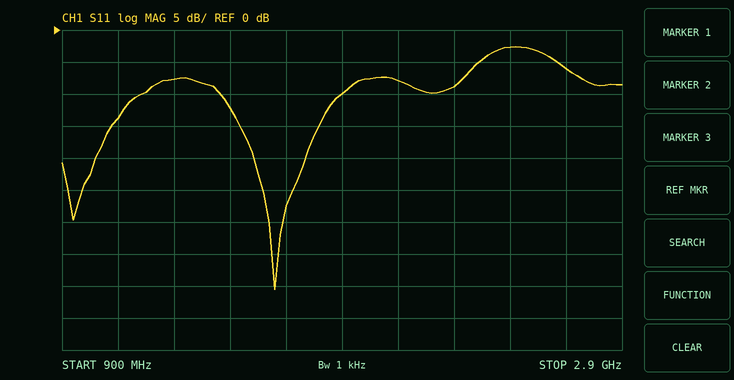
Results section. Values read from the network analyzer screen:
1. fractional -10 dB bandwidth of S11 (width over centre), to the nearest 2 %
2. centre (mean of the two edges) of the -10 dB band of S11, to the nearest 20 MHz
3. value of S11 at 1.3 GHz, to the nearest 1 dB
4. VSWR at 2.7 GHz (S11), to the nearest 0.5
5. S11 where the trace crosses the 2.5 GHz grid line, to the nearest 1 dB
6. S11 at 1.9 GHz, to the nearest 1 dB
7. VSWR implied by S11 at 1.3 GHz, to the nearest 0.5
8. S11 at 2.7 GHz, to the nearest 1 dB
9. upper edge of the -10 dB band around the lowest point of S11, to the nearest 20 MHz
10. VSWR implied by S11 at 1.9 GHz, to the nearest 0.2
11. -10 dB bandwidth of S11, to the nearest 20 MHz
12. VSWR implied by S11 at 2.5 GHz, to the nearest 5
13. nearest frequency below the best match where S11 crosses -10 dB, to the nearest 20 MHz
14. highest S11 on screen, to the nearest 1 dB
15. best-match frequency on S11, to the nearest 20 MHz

26 %
1.68 GHz
-8 dB
3.0
-3 dB
-10 dB
2.5
-6 dB
1.90 GHz
2.0
440 MHz
5
1.46 GHz
-3 dB
1.66 GHz
